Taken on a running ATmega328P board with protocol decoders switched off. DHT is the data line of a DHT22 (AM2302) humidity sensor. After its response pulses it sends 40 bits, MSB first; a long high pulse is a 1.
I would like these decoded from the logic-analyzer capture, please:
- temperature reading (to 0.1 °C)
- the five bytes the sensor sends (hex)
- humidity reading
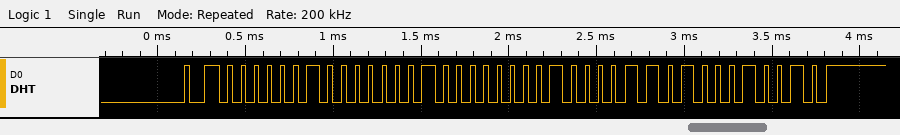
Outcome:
26.9 °C
02 02 01 0D 12
51.4 %
